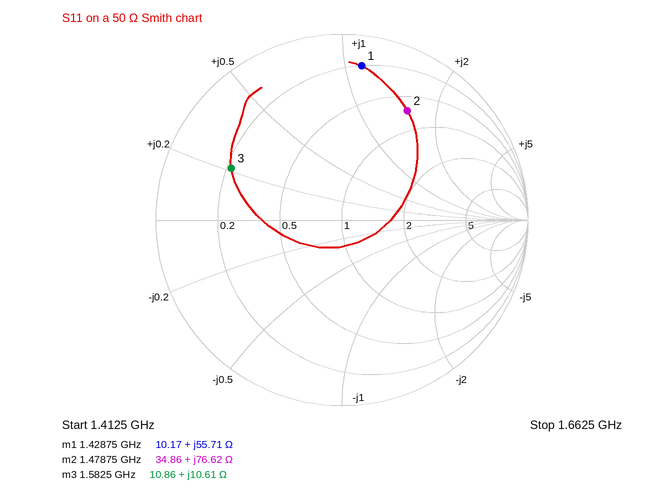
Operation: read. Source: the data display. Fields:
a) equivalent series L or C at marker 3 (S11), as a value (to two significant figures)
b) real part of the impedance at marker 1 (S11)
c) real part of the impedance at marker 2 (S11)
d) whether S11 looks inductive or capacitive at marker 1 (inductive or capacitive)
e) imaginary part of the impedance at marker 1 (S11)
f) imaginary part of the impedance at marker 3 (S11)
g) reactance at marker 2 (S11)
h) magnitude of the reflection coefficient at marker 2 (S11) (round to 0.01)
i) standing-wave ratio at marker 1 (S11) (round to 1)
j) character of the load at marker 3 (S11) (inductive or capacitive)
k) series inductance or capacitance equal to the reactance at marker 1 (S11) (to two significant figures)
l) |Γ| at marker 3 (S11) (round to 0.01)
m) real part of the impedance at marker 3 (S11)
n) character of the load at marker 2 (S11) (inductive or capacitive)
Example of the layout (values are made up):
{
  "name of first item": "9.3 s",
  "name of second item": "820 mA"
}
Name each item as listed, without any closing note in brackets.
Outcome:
{
  "equivalent series L or C at marker 3 (S11), as a value": "1.1 nH",
  "real part of the impedance at marker 1": "10.17 Ω",
  "real part of the impedance at marker 2": "34.86 Ω",
  "whether S11 looks inductive or capacitive at marker 1": "inductive",
  "imaginary part of the impedance at marker 1": "+55.71 Ω",
  "imaginary part of the impedance at marker 3": "+10.61 Ω",
  "reactance at marker 2": "+76.62 Ω",
  "magnitude of the reflection coefficient at marker 2 (S11)": "0.68",
  "standing-wave ratio at marker 1 (S11)": "11",
  "character of the load at marker 3 (S11)": "inductive",
  "series inductance or capacitance equal to the reactance at marker 1 (S11)": "6.2 nH",
  "|Γ| at marker 3 (S11)": "0.66",
  "real part of the impedance at marker 3": "10.86 Ω",
  "character of the load at marker 2 (S11)": "inductive"
}
